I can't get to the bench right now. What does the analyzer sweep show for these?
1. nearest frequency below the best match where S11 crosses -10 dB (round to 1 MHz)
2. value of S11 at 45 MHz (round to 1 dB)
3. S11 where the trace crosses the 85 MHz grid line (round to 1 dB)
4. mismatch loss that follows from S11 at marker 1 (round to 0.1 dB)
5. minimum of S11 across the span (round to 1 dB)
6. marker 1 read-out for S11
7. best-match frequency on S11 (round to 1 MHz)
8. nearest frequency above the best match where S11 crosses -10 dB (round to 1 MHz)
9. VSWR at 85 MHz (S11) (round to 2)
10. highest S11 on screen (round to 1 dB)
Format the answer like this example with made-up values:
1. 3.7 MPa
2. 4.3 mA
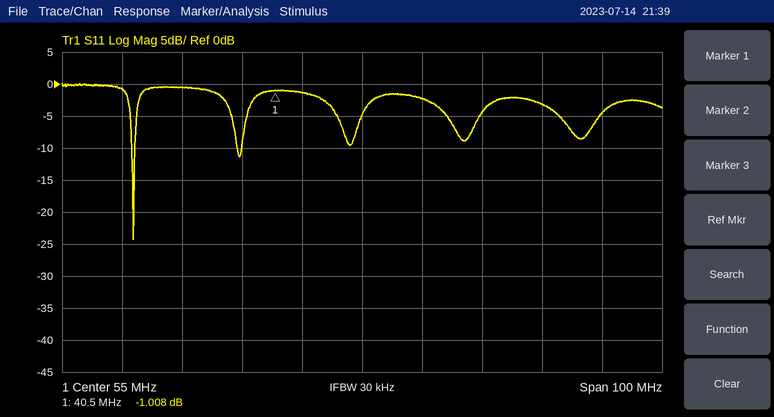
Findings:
1. 17 MHz
2. -1 dB
3. -3 dB
4. 6.8 dB
5. -24 dB
6. -1.008 dB
7. 17 MHz
8. 17 MHz
9. 6
10. 0 dB
